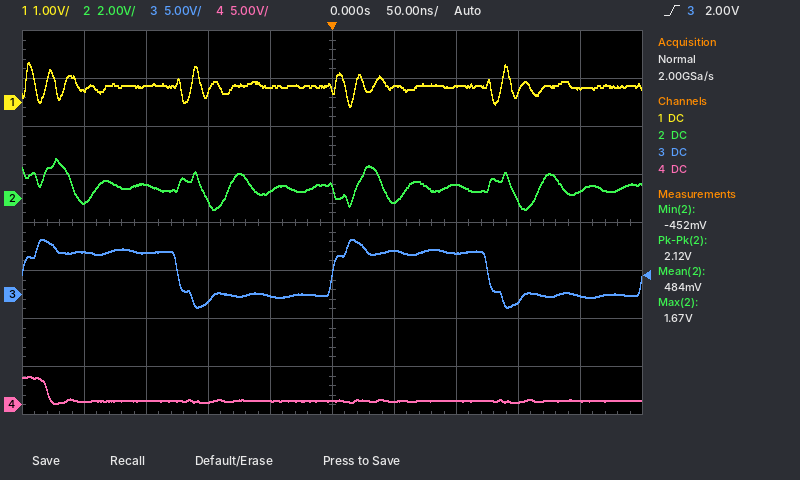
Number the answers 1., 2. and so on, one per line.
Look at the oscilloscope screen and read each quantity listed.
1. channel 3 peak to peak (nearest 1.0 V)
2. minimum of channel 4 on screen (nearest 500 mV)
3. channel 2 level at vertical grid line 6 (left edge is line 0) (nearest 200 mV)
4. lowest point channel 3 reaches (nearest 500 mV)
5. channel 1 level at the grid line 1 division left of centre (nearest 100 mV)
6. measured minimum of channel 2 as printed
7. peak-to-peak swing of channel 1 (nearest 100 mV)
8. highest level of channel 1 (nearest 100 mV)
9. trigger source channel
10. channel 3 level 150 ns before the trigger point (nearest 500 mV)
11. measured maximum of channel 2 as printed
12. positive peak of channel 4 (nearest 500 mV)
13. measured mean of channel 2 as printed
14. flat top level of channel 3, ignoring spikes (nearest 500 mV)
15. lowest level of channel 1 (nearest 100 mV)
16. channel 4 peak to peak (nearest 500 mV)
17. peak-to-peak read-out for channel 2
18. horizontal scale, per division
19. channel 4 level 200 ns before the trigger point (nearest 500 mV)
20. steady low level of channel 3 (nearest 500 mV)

1. 7.0 V
2. 0.0 V
3. -200 mV
4. -1.5 V
5. 300 mV
6. -452 mV
7. 900 mV
8. 800 mV
9. channel 3
10. 4.5 V
11. 1.67 V
12. 3.0 V
13. 484 mV
14. 4.5 V
15. -100 mV
16. 3.0 V
17. 2.12 V
18. 50 ns
19. 500 mV
20. 0.0 V
